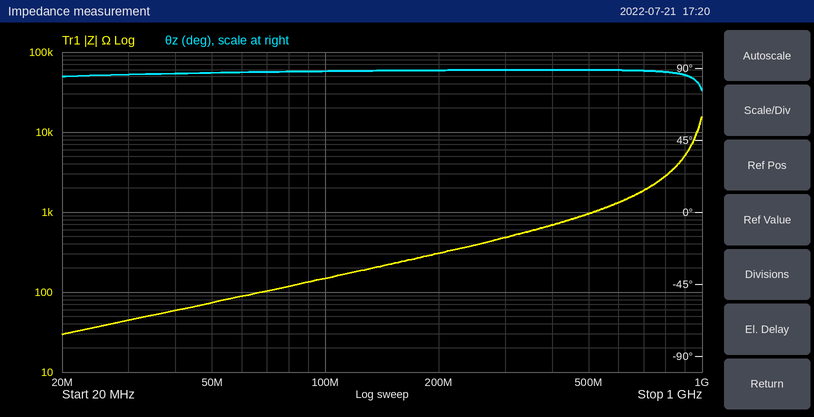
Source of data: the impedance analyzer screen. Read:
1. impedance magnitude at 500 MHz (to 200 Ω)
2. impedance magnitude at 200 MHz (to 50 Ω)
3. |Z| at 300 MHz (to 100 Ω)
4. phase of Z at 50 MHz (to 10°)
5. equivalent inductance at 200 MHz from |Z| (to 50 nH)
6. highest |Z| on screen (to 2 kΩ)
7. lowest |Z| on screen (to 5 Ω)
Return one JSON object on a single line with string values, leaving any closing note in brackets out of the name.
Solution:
{"impedance magnitude at 500 MHz": "1.0 kΩ", "impedance magnitude at 200 MHz": "300 Ω", "|Z| at 300 MHz": "500 Ω", "phase of Z at 50 MHz": "90°", "equivalent inductance at 200 MHz from |Z|": "250 nH", "highest |Z| on screen": "16 kΩ", "lowest |Z| on screen": "30 Ω"}
